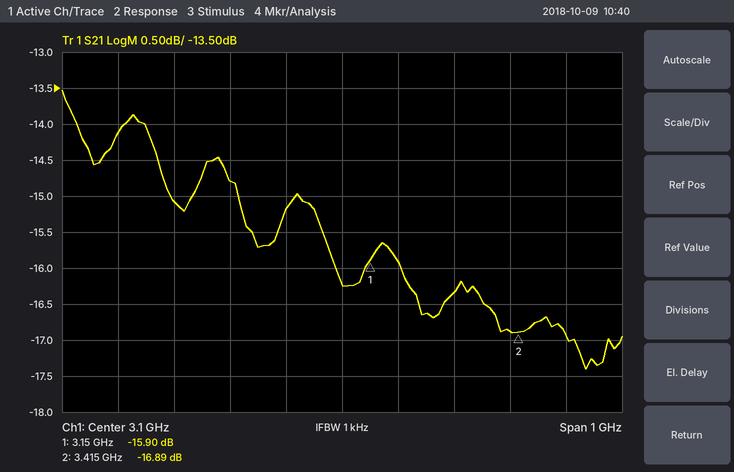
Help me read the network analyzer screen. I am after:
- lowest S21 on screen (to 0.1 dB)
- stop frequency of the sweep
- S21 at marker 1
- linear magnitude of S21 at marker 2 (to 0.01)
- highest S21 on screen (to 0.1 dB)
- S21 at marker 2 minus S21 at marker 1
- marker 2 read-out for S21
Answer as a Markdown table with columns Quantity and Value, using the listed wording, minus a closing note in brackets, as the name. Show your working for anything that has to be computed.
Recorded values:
| Quantity | Value |
|---|---|
| lowest S21 on screen | -17.4 dB |
| stop frequency of the sweep | 3.6 GHz |
| S21 at marker 1 | -15.90 dB |
| linear magnitude of S21 at marker 2 | 10^(-16.89/20) ≈ 0.14 |
| highest S21 on screen | -13.5 dB |
| S21 at marker 2 minus S21 at marker 1 | -16.89 − (-15.9) = -0.99 dB |
| marker 2 read-out for S21 | -16.89 dB |
